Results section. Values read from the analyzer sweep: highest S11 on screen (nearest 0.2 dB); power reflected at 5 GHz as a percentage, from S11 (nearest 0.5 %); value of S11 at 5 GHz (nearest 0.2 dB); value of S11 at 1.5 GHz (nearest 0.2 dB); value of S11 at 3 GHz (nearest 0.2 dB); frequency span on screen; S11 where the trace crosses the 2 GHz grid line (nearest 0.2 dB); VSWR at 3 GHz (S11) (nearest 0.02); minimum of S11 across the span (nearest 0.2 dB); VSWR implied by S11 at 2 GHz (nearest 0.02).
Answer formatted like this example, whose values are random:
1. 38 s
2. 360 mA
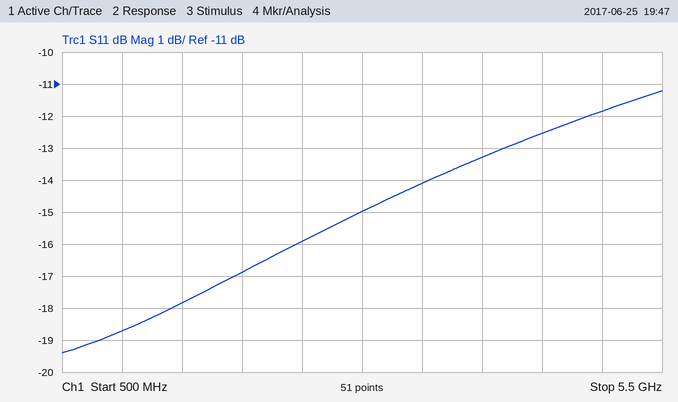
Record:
1. -11.2 dB
2. 6.5 %
3. -11.8 dB
4. -17.8 dB
5. -15.0 dB
6. 5 GHz
7. -16.8 dB
8. 1.44
9. -19.4 dB
10. 1.34
